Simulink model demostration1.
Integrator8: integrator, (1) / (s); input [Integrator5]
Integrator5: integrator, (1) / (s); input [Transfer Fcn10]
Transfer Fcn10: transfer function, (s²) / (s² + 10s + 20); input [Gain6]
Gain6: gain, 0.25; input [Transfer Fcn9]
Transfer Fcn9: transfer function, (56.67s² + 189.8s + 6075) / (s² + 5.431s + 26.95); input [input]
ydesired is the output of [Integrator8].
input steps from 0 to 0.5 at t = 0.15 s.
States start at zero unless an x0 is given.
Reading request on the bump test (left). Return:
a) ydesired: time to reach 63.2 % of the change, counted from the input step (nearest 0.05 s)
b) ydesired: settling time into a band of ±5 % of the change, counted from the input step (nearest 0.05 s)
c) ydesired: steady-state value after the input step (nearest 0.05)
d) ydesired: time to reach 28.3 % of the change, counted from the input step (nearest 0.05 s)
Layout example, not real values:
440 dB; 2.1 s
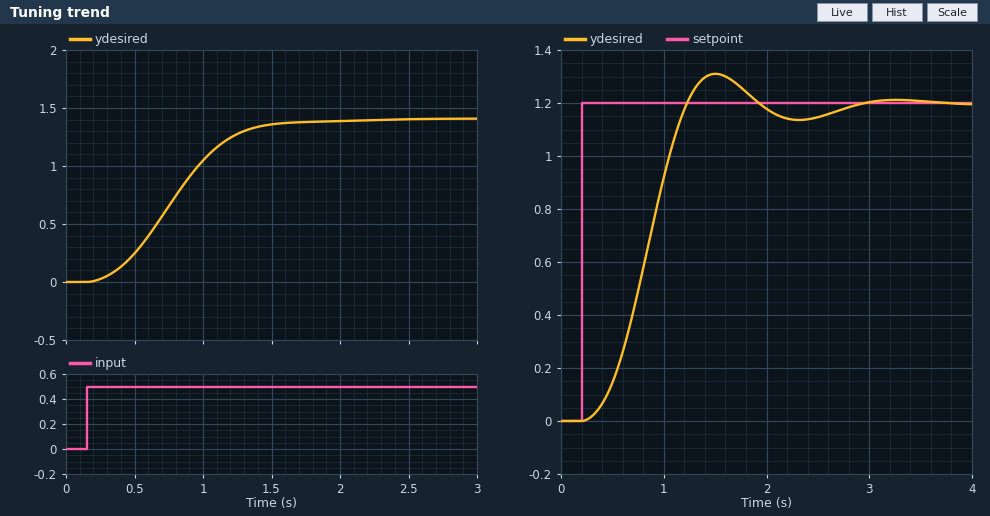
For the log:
0.75 s; 1.25 s; 1.40; 0.45 s
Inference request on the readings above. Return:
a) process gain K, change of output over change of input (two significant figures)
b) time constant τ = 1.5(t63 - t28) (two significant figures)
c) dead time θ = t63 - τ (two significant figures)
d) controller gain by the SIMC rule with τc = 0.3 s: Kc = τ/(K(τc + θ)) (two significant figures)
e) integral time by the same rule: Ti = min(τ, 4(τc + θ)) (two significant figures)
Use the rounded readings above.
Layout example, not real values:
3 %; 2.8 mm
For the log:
2.8; 0.45 s; 0.30 s; 0.27; 0.45 s
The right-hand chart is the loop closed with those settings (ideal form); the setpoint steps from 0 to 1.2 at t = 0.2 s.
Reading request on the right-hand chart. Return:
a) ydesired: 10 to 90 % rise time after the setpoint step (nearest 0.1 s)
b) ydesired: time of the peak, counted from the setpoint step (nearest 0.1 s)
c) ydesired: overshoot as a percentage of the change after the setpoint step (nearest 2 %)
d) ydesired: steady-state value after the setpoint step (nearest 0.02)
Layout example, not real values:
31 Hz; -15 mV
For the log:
0.6 s; 1.3 s; 10 %; 1.20
